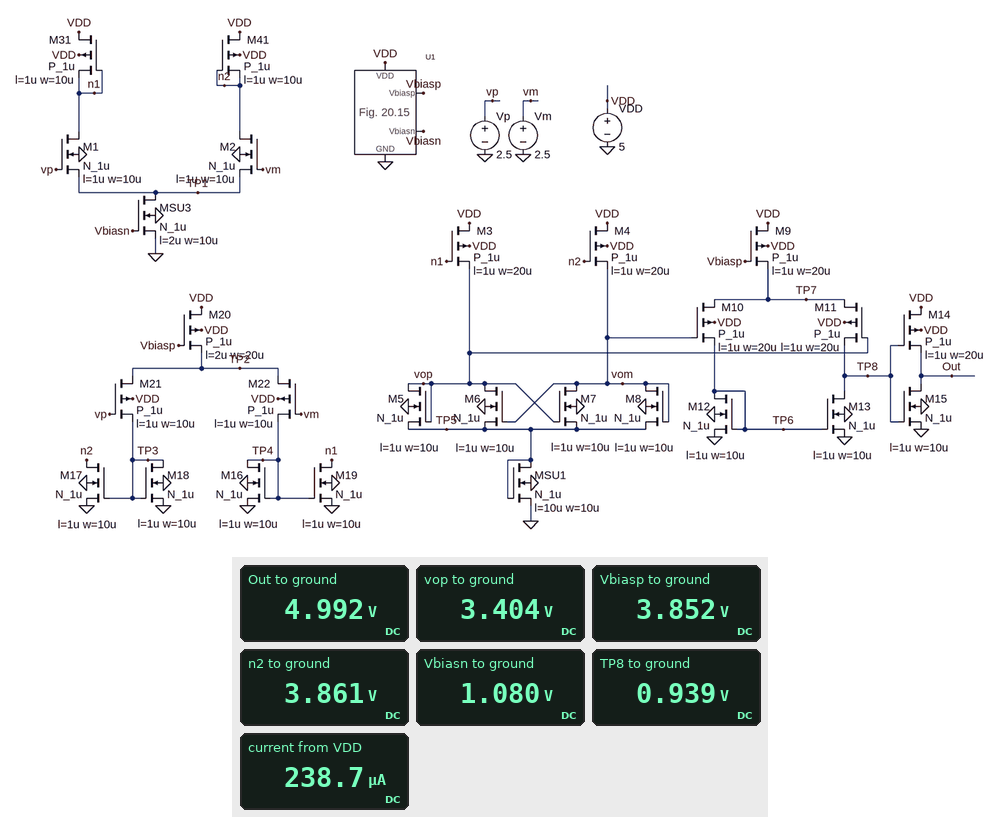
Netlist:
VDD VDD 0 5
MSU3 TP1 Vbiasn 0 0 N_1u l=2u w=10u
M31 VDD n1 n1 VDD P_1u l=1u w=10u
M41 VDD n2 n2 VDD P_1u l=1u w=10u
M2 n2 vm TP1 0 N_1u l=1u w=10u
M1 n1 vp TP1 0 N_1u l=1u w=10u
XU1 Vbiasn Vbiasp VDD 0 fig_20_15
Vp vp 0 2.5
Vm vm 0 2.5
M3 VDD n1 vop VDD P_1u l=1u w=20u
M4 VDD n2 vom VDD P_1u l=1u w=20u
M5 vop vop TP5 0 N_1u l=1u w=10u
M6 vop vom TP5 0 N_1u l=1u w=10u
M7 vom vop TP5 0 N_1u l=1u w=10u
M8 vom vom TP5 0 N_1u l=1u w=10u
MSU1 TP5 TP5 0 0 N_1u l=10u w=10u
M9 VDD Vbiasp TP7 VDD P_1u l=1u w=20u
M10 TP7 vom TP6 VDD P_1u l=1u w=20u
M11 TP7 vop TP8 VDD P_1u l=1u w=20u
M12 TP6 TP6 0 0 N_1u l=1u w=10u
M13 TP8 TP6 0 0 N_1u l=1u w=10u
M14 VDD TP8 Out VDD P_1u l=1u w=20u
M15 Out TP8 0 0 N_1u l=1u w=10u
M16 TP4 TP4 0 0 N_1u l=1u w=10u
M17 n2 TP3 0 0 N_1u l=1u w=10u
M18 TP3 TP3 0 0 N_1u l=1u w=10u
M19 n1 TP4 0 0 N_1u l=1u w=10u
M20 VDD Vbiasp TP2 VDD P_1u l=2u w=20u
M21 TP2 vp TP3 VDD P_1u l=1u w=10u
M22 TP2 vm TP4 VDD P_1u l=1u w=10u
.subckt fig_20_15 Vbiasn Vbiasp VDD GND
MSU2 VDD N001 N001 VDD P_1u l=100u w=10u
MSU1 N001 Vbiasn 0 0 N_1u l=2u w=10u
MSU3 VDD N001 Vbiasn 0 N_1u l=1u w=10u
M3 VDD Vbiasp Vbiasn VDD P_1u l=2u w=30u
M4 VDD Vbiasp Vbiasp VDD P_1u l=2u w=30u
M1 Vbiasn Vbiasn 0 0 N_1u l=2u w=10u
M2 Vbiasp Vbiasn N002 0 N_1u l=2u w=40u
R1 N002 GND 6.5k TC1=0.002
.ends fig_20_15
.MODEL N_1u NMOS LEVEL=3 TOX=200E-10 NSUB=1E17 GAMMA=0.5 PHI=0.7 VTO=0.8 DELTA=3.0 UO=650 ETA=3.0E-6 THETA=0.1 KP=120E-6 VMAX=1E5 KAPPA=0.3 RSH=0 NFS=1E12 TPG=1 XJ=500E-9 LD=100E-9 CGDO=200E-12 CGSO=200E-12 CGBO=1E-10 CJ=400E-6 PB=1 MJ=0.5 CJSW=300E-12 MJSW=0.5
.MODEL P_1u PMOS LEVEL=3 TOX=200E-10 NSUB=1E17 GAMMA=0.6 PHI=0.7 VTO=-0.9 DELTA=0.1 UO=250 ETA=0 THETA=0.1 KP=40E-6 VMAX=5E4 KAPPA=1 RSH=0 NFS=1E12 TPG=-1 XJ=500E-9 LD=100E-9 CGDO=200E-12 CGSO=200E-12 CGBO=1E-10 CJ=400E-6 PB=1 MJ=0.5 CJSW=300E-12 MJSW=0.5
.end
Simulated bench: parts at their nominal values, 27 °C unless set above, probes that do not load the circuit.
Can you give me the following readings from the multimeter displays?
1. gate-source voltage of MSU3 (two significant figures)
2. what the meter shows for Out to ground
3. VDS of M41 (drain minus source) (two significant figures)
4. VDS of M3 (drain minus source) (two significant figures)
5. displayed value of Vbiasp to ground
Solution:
1.1 V
4.992 V
1.1 V
1.6 V
3.852 V
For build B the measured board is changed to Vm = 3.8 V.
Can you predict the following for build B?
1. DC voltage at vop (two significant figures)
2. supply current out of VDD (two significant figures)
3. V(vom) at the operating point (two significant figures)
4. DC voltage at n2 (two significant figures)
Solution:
2.1 V
220 µA
3.6 V
3.7 V
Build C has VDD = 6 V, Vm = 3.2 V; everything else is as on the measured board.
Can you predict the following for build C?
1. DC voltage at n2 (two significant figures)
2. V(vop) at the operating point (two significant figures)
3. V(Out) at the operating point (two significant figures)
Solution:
4.7 V
2.2 V
7.0 mV
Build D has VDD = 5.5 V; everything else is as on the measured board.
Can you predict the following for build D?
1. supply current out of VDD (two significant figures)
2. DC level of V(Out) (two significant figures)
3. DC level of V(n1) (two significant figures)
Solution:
250 µA
5.5 V
4.4 V
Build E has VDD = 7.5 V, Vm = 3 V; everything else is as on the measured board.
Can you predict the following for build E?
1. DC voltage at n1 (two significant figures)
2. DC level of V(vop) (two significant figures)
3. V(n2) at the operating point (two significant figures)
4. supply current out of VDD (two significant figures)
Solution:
6.9 V
2.3 V
6.2 V
950 µA
